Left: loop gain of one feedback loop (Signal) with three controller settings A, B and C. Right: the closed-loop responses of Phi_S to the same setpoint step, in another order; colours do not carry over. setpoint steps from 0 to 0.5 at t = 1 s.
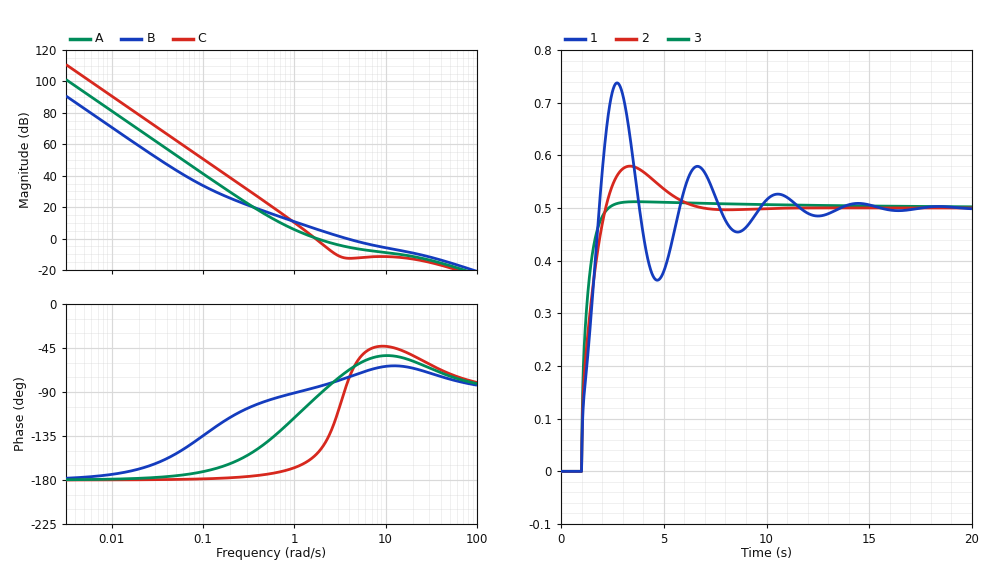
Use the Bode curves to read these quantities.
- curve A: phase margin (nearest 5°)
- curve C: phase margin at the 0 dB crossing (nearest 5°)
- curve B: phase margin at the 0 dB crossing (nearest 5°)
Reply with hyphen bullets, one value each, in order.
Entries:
- 85°
- 25°
- 105°
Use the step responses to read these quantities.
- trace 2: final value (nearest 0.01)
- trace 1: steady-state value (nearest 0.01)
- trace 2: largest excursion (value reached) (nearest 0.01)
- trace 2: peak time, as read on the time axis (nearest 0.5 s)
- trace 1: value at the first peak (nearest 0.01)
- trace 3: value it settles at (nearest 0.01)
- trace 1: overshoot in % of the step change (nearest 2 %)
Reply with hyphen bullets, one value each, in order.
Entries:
- 0.50
- 0.50
- 0.58
- 3.5 s
- 0.74
- 0.50
- 48 %
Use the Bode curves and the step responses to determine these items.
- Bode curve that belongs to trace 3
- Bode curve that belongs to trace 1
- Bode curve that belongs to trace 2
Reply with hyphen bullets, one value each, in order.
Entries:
- B
- C
- A
